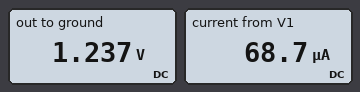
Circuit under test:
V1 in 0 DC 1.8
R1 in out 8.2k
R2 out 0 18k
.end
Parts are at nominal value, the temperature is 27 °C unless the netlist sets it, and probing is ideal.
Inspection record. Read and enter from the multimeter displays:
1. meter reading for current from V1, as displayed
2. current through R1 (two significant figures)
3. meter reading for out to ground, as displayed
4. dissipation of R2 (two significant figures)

68.7 µA
69 µA
1.237 V
85 µW
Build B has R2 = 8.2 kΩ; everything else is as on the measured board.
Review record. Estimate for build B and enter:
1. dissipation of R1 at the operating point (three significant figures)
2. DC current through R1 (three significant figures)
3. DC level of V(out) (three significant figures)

98.8 µW
110 µA
900 mV
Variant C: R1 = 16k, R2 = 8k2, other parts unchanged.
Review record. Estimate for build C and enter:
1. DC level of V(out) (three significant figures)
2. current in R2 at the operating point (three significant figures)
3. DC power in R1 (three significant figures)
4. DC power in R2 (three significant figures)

610 mV
74.4 µA
88.5 µW
45.4 µW
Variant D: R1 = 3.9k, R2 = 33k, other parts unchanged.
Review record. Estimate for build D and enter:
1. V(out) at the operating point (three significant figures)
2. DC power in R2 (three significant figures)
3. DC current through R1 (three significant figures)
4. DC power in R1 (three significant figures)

1.61 V
78.5 µW
48.8 µA
9.28 µW
